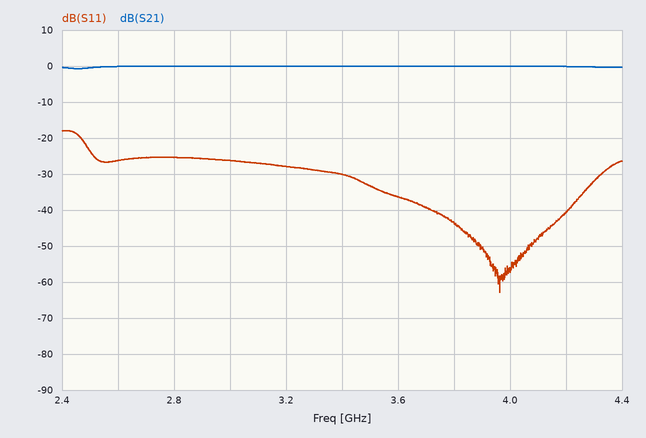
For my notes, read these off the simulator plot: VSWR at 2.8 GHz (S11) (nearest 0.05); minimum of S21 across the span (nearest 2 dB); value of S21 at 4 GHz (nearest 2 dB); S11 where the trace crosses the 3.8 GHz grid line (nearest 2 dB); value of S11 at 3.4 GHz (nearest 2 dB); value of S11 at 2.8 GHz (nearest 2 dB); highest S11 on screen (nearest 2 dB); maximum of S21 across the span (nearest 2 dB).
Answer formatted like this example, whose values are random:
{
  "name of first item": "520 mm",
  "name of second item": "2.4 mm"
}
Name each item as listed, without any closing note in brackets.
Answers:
{
  "VSWR at 2.8 GHz (S11)": "1.10",
  "minimum of S21 across the span": "0 dB",
  "value of S21 at 4 GHz": "0 dB",
  "S11 where the trace crosses the 3.8 GHz grid line": "-44 dB",
  "value of S11 at 3.4 GHz": "-30 dB",
  "value of S11 at 2.8 GHz": "-26 dB",
  "highest S11 on screen": "-18 dB",
  "maximum of S21 across the span": "0 dB"
}
